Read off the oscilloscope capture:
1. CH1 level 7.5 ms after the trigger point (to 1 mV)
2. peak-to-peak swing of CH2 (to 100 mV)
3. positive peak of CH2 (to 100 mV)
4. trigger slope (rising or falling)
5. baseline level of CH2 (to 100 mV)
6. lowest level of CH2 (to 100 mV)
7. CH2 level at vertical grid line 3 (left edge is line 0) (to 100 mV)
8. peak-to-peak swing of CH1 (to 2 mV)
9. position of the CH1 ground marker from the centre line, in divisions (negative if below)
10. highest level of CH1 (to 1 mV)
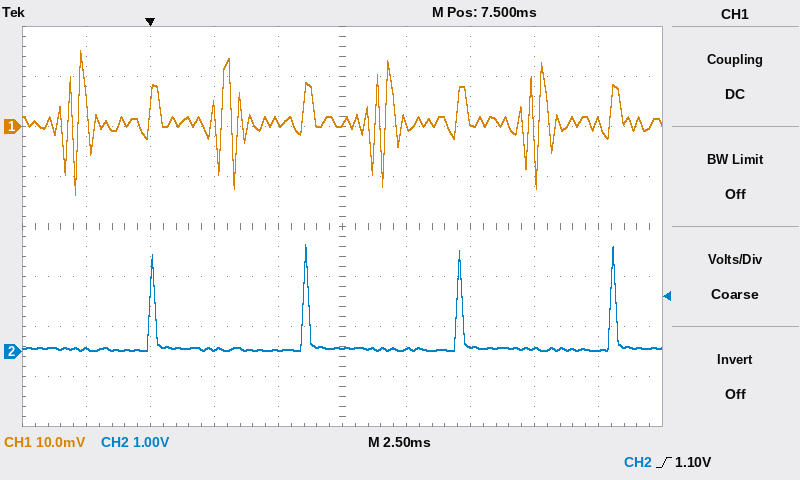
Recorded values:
1 mV
2.1 V
2.1 V
rising
100 mV
0.0 V
0.0 V
28 mV
+2.0 div
15 mV
